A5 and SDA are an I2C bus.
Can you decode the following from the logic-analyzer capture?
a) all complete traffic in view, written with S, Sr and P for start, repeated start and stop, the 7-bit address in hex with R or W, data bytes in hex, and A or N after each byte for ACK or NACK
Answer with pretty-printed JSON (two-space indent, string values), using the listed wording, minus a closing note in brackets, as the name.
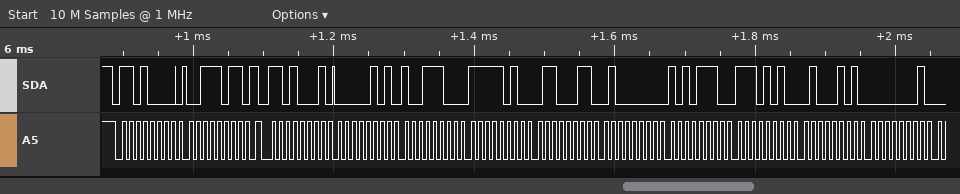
{
  "all complete traffic in view, written with S, Sr and P for start, repeated start and stop, the 7-bit address in hex with R or W, data bytes in hex, and A or N after each byte for ACK or NACK": "S 68W A 3B A Sr 68R A 05 A 9C A FA A 63 A 40 A AE A EA A 45 A 01 A"
}
